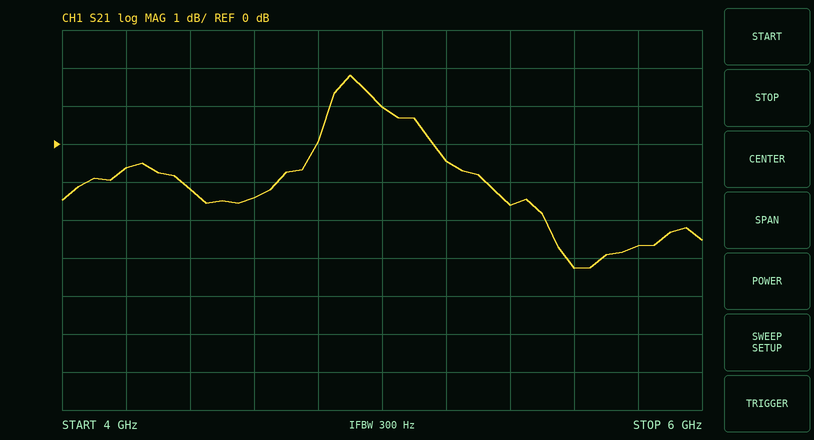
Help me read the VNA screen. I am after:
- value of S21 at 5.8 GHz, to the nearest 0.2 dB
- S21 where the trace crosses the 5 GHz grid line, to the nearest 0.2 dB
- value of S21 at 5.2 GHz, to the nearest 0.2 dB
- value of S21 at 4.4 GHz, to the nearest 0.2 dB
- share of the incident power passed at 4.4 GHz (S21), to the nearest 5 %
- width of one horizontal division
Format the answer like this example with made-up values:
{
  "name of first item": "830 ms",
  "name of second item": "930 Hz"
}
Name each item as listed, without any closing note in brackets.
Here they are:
{
  "value of S21 at 5.8 GHz, to the nearest 0.2 dB": "-2.6 dB",
  "S21 where the trace crosses the 5 GHz grid line, to the nearest 0.2 dB": "1.0 dB",
  "value of S21 at 5.2 GHz, to the nearest 0.2 dB": "-0.4 dB",
  "value of S21 at 4.4 GHz, to the nearest 0.2 dB": "-1.2 dB",
  "share of the incident power passed at 4.4 GHz (S21), to the nearest 5 %": "75 %",
  "width of one horizontal division": "200 MHz"
}
